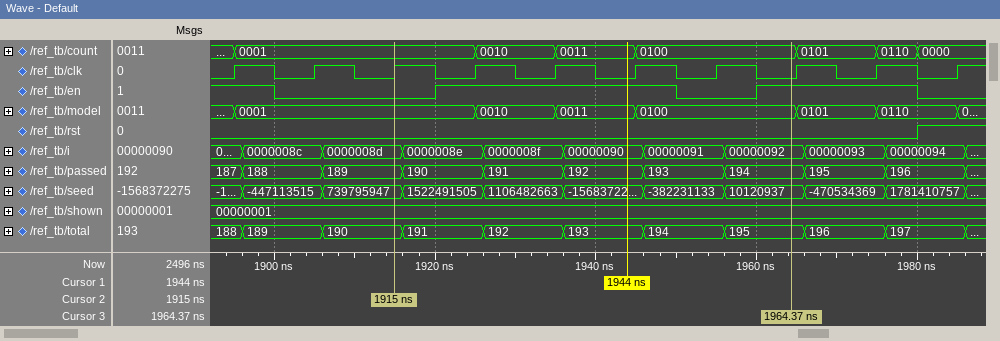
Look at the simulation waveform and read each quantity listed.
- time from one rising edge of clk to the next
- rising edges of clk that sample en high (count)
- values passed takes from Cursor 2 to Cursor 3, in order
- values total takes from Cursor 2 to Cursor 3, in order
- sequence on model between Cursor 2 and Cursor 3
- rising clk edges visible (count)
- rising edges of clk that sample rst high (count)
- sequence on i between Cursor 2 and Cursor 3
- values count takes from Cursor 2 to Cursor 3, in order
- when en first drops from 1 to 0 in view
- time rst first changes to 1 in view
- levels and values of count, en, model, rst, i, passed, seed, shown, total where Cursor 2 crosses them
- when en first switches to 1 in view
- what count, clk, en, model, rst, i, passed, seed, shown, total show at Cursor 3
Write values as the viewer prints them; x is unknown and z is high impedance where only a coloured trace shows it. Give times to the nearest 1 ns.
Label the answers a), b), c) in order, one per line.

a) 10 ns
b) 6
c) 189, 190, 191, 192, 193, 194
d) 190, 191, 192, 193, 194, 195
e) 0001, 0010, 0011, 0100
f) 10
g) 1
h) 0000008d, 0000008e, 0000008f, 00000090, 00000091, 00000092
i) 0001, 0010, 0011, 0100
j) 1900 ns
k) 1980 ns
l) count=0001, en=0, model=0001, rst=0, i=0000008d, passed=189, seed=739795947, shown=00000001, total=190
m) 1920 ns
n) count=0100, clk=0, en=1, model=0100, rst=0, i=00000092, passed=194, seed=10120937, shown=00000001, total=195
